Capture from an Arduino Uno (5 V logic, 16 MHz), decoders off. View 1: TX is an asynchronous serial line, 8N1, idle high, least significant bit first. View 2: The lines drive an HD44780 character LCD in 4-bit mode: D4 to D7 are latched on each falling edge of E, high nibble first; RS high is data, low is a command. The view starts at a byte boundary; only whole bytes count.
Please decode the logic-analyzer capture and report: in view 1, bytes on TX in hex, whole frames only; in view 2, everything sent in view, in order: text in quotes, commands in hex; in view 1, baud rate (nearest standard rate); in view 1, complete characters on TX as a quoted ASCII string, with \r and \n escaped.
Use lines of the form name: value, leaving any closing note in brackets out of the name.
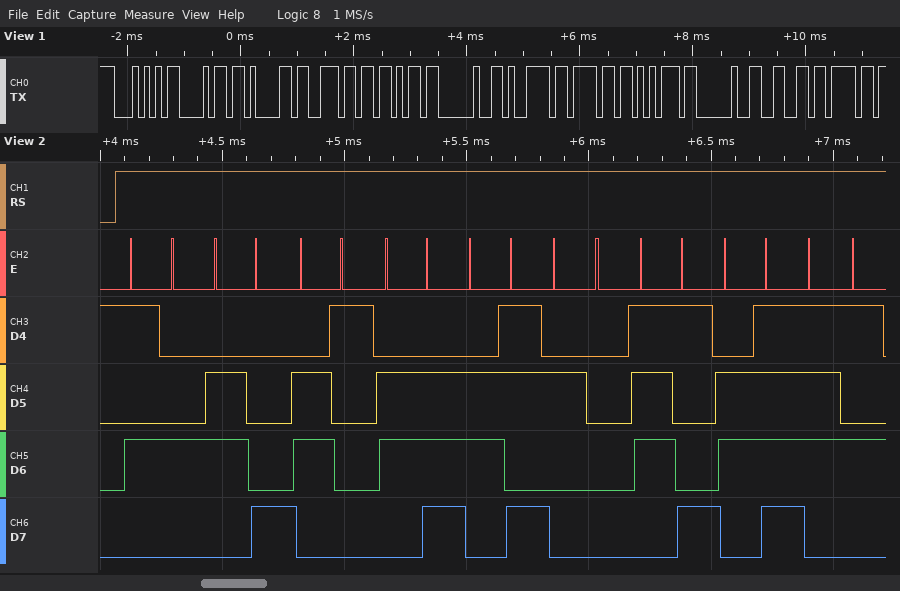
in view 1, bytes on TX in hex, whole frames only: 54 68 61 6E 6B 20 79 6F 75 20 66 6F
in view 2, everything sent in view, in order: text in quotes, commands in hex: "Thank you"
in view 1, baud rate: 9600 baud
in view 1, complete characters on TX as a quoted ASCII string, with \r and \n escaped: "Thank you fo"
